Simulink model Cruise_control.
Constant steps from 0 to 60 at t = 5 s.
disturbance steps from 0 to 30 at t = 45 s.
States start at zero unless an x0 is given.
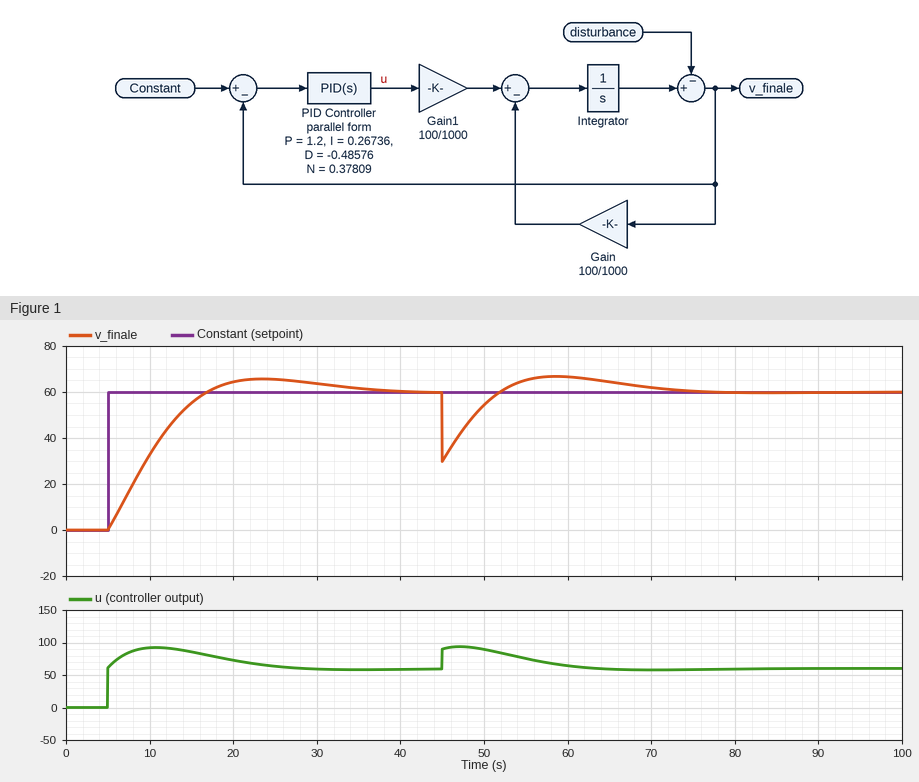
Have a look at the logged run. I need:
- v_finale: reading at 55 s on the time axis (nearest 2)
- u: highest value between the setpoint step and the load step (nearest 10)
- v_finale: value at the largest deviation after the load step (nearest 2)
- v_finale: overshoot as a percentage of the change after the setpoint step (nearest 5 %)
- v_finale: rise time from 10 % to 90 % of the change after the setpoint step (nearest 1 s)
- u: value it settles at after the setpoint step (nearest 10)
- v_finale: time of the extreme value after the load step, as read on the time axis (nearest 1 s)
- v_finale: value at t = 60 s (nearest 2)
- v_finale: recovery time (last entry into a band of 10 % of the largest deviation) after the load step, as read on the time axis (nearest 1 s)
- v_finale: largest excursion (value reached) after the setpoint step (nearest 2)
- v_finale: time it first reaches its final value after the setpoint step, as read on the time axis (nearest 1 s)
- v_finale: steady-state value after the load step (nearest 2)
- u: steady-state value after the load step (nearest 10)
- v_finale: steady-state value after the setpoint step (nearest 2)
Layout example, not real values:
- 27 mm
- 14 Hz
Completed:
- 66
- 90
- 30
- 10 %
- 9 s
- 60
- 45 s
- 66
- 68 s
- 66
- 17 s
- 60
- 60
- 60
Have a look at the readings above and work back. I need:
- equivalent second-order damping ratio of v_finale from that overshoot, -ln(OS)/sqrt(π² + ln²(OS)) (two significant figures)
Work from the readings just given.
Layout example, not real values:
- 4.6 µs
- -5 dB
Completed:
- 0.59
